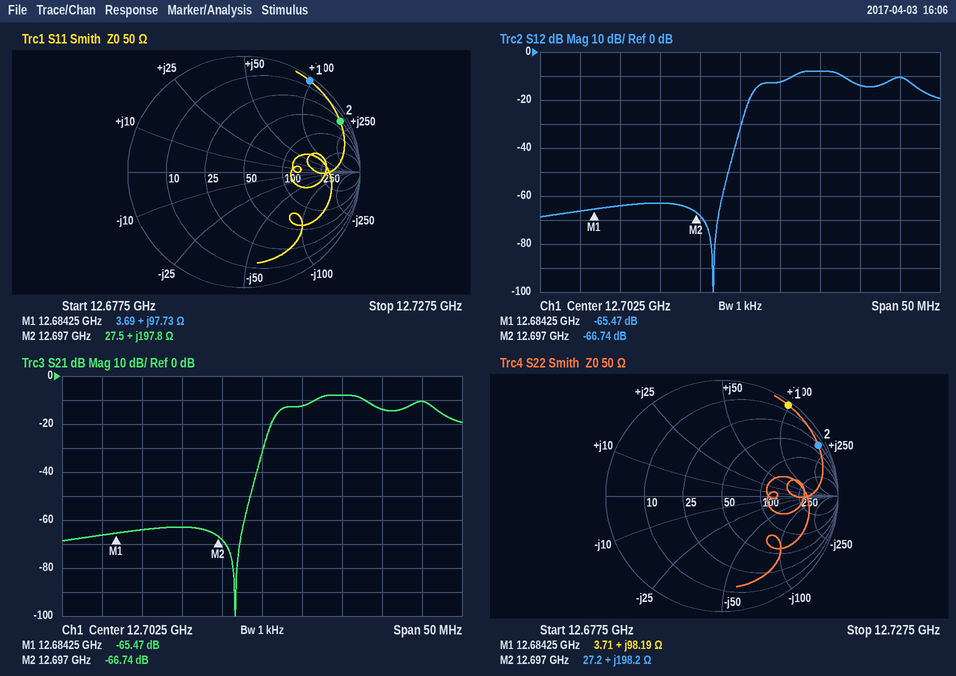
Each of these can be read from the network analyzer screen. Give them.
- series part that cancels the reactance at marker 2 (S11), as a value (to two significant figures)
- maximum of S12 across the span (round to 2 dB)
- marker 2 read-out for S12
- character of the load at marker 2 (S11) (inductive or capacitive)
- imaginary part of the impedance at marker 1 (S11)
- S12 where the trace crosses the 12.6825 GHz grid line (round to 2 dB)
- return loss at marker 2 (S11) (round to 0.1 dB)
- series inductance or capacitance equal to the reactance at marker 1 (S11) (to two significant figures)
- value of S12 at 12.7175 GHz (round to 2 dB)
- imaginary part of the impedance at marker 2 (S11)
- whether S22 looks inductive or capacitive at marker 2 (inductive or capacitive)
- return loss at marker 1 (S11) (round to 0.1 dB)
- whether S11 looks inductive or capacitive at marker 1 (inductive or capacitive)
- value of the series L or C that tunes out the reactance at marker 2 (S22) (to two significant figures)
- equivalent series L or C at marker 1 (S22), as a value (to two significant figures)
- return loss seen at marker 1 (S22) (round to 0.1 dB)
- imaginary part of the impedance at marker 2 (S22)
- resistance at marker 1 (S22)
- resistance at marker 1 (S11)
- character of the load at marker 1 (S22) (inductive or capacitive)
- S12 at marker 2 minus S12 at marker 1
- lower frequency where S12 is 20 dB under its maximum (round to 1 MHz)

63 fF
-8 dB
-66.74 dB
inductive
+97.73 Ω
-66 dB
0.6 dB
1.2 nH
-14 dB
+197.8 Ω
inductive
0.3 dB
inductive
63 fF
1.2 nH
0.3 dB
+198.2 Ω
3.71 Ω
3.69 Ω
inductive
-1.27 dB
12.703 GHz
